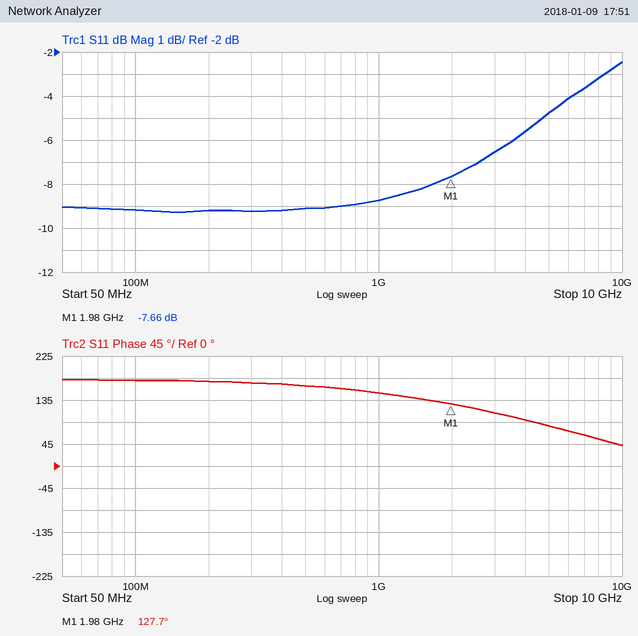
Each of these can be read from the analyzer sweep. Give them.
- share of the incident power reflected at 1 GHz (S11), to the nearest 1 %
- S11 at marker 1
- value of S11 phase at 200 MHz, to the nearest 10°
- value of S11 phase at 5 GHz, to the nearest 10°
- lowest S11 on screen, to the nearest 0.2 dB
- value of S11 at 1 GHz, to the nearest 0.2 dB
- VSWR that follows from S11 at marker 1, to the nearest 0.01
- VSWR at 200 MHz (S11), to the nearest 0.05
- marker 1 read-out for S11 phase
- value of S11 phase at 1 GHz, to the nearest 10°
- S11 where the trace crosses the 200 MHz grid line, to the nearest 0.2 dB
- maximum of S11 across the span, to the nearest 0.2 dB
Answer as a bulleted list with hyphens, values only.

- 13 %
- -7.66 dB
- 170°
- 80°
- -9.2 dB
- -8.8 dB
- 2.41
- 2.05
- 127.7°
- 150°
- -9.2 dB
- -2.4 dB
